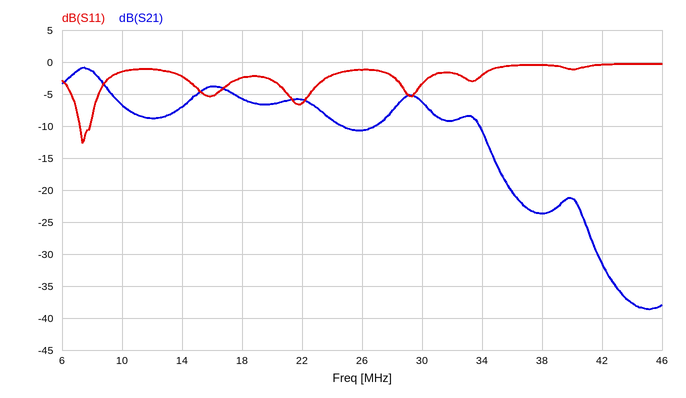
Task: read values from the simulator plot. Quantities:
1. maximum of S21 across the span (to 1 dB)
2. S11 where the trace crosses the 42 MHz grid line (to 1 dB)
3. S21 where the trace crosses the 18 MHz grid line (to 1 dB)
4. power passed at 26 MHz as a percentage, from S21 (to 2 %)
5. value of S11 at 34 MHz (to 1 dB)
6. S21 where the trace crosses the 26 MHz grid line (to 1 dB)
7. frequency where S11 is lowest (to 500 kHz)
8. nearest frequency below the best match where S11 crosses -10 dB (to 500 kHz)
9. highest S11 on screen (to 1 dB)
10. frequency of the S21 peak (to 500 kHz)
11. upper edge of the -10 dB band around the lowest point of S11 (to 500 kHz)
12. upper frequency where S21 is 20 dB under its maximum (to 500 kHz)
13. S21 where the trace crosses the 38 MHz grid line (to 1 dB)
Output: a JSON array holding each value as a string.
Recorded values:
["-1 dB", "0 dB", "-6 dB", "8 %", "-2 dB", "-11 dB", "7.5 MHz", "7.0 MHz", "0 dB", "7.5 MHz", "8.0 MHz", "36.0 MHz", "-24 dB"]
